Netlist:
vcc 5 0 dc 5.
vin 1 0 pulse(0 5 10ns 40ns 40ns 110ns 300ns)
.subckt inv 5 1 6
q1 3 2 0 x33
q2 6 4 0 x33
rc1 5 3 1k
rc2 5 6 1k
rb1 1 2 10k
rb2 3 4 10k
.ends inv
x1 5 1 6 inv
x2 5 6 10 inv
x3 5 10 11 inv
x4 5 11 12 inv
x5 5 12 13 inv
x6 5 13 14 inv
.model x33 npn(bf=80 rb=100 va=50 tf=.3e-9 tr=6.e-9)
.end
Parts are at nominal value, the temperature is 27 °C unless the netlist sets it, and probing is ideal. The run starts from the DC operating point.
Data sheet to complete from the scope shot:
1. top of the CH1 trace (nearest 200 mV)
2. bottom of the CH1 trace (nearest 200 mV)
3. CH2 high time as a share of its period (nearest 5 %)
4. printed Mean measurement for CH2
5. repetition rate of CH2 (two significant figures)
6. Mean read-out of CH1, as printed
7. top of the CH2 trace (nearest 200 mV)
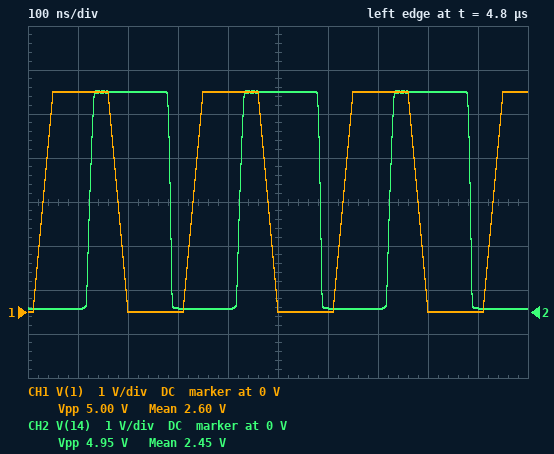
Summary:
5.0 V
0 V
55 %
2.45 V
3.3 MHz
2.60 V
5.0 V
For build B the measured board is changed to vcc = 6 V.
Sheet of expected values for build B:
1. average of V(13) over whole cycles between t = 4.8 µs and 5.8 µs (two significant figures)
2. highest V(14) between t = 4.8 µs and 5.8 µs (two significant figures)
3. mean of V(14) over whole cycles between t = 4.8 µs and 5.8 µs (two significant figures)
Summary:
2.9 V
6.0 V
3.2 V
